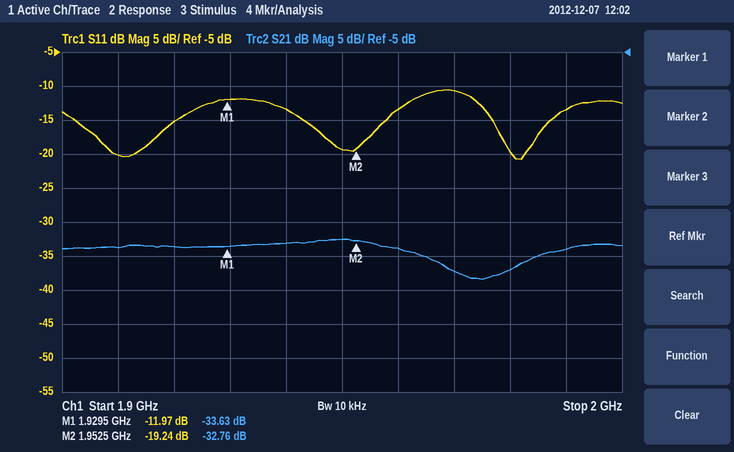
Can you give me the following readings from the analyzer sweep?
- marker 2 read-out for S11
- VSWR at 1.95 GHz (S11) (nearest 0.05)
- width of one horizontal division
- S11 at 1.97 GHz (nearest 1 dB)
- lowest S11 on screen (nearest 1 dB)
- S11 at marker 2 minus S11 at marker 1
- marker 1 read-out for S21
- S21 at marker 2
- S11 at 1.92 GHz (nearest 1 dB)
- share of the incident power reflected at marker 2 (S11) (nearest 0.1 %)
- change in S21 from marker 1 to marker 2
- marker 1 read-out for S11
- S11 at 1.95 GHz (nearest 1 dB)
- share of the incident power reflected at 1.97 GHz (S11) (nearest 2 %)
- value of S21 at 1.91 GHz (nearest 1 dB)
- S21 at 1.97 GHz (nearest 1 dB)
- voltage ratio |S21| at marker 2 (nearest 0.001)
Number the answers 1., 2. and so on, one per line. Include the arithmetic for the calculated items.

1. -19.24 dB
2. |Γ| = 10^(-19/20) = 0.1122; VSWR = (1 + 0.1122)/(1 − 0.1122) ≈ 1.25
3. 10 MHz
4. -11 dB
5. -21 dB
6. -19.24 − (-11.97) = -7.27 dB
7. -33.63 dB
8. -32.76 dB
9. -15 dB
10. 10^(-19.24/10) ≈ 1.2 %
11. -32.76 − (-33.63) = 0.87 dB
12. -11.97 dB
13. -19 dB
14. 10^(-11/10) ≈ 8 %
15. -34 dB
16. -37 dB
17. 10^(-32.76/20) ≈ 0.023
